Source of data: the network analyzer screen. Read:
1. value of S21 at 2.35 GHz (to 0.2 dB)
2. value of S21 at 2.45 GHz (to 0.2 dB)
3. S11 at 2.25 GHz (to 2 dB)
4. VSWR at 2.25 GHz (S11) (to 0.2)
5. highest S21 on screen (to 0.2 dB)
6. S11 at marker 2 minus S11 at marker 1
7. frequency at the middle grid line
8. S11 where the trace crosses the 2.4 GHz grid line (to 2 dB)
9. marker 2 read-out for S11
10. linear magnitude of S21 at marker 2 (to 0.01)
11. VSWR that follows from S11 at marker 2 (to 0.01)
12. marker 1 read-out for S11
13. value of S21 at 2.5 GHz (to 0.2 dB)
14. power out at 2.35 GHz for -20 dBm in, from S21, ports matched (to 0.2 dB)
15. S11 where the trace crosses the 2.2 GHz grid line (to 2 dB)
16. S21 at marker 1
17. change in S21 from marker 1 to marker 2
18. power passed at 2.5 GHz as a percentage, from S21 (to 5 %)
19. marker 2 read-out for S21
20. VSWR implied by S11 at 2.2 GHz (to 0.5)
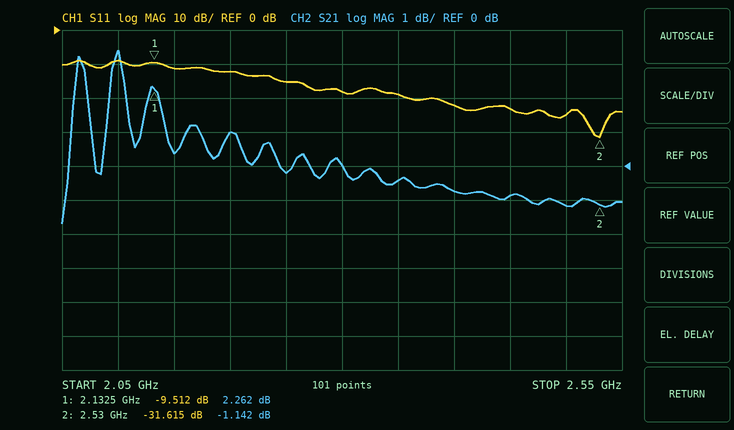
-0.4 dB
-0.8 dB
-16 dB
1.4
3.4 dB
-22.103 dB
2.3 GHz
-22 dB
-31.615 dB
0.88
1.05
-9.512 dB
-1.2 dB
-20.4 dBm
-12 dB
2.262 dB
-3.404 dB
75 %
-1.142 dB
1.5
